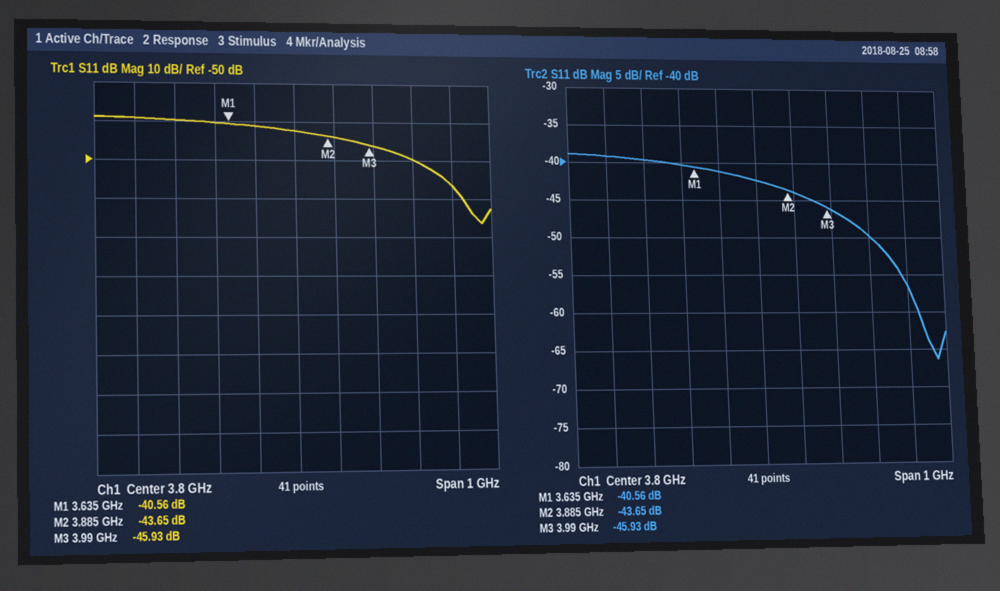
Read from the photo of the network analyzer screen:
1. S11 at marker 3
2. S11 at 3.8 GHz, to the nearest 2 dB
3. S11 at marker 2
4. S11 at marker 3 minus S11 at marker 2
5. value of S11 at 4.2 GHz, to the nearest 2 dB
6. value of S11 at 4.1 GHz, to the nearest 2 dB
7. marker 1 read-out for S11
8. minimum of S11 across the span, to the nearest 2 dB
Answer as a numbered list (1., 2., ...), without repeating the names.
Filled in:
1. -45.93 dB
2. -42 dB
3. -43.65 dB
4. -2.28 dB
5. -56 dB
6. -50 dB
7. -40.56 dB
8. -66 dB
